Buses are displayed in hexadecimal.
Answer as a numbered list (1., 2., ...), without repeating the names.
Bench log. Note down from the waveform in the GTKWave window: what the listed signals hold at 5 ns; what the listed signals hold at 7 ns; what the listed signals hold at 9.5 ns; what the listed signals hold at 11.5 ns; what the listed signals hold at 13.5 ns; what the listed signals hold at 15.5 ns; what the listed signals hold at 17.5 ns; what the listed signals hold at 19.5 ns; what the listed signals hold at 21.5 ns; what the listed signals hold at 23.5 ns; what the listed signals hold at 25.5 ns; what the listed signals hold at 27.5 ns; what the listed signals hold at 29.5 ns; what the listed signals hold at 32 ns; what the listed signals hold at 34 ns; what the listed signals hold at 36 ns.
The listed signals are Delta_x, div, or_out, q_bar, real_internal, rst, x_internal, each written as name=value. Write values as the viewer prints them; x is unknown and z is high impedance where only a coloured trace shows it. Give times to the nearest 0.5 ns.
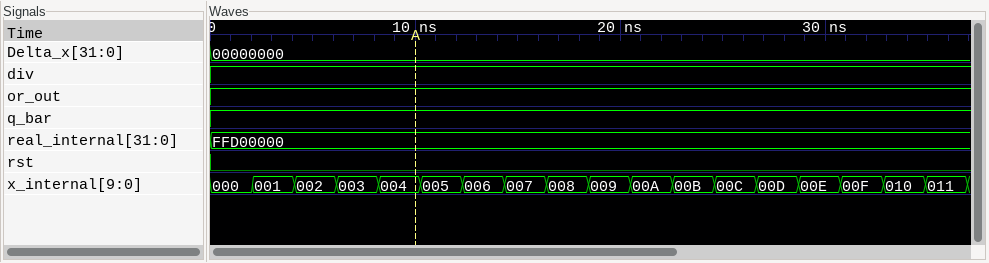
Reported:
1. Delta_x=00000000, div=1, or_out=1, q_bar=1, real_internal=FFD00000, rst=0, x_internal=002
2. Delta_x=00000000, div=1, or_out=1, q_bar=1, real_internal=FFD00000, rst=0, x_internal=003
3. Delta_x=00000000, div=1, or_out=1, q_bar=1, real_internal=FFD00000, rst=0, x_internal=004
4. Delta_x=00000000, div=1, or_out=1, q_bar=1, real_internal=FFD00000, rst=0, x_internal=005
5. Delta_x=00000000, div=1, or_out=1, q_bar=1, real_internal=FFD00000, rst=0, x_internal=006
6. Delta_x=00000000, div=1, or_out=1, q_bar=1, real_internal=FFD00000, rst=0, x_internal=007
7. Delta_x=00000000, div=1, or_out=1, q_bar=1, real_internal=FFD00000, rst=0, x_internal=008
8. Delta_x=00000000, div=1, or_out=1, q_bar=1, real_internal=FFD00000, rst=0, x_internal=009
9. Delta_x=00000000, div=1, or_out=1, q_bar=1, real_internal=FFD00000, rst=0, x_internal=00A
10. Delta_x=00000000, div=1, or_out=1, q_bar=1, real_internal=FFD00000, rst=0, x_internal=00B
11. Delta_x=00000000, div=1, or_out=1, q_bar=1, real_internal=FFD00000, rst=0, x_internal=00C
12. Delta_x=00000000, div=1, or_out=1, q_bar=1, real_internal=FFD00000, rst=0, x_internal=00D
13. Delta_x=00000000, div=1, or_out=1, q_bar=1, real_internal=FFD00000, rst=0, x_internal=00E
14. Delta_x=00000000, div=1, or_out=1, q_bar=1, real_internal=FFD00000, rst=0, x_internal=00F
15. Delta_x=00000000, div=1, or_out=1, q_bar=1, real_internal=FFD00000, rst=0, x_internal=010
16. Delta_x=00000000, div=1, or_out=1, q_bar=1, real_internal=FFD00000, rst=0, x_internal=011
